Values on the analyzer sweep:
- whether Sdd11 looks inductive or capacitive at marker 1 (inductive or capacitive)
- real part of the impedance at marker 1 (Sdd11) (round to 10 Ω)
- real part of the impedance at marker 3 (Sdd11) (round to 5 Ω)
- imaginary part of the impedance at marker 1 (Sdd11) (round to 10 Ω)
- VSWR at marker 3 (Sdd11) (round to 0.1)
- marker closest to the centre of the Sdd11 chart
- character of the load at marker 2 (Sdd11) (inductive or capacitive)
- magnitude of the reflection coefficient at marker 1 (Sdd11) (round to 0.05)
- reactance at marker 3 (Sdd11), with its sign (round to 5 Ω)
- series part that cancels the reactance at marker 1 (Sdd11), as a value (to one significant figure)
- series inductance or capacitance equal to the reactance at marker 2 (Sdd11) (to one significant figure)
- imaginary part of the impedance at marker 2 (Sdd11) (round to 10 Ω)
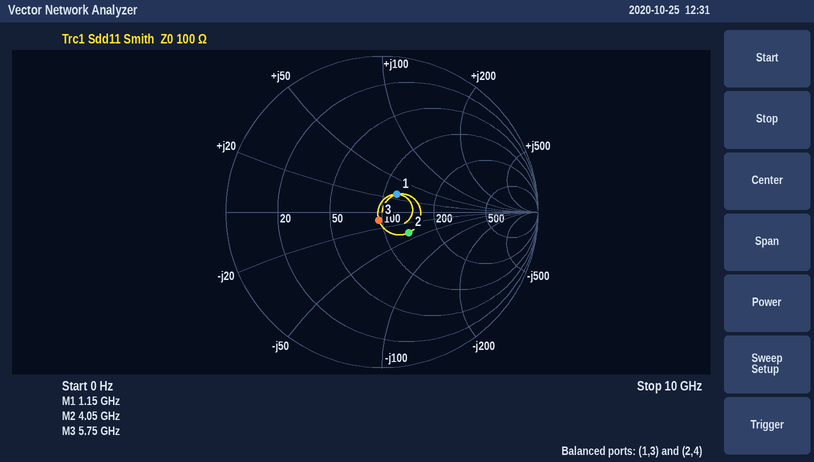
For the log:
inductive
120 Ω
95 Ω
+30 Ω
1.1
marker 3
capacitive
0.15
-10 Ω
5 pF
1 pF
-40 Ω
